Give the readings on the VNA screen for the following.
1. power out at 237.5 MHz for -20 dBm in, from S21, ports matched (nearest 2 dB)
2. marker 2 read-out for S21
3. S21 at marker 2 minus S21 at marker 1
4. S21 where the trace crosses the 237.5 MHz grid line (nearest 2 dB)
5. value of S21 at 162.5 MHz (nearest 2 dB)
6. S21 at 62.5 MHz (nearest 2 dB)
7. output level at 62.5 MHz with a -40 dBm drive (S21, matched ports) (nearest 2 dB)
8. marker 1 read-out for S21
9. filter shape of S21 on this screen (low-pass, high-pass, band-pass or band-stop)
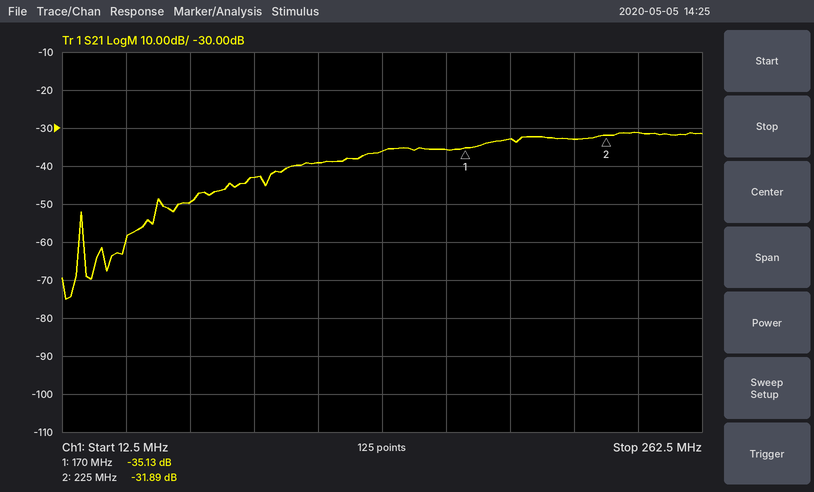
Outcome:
-52 dBm
-31.89 dB
3.24 dB
-32 dB
-36 dB
-50 dB
-90 dBm
-35.13 dB
high-pass
